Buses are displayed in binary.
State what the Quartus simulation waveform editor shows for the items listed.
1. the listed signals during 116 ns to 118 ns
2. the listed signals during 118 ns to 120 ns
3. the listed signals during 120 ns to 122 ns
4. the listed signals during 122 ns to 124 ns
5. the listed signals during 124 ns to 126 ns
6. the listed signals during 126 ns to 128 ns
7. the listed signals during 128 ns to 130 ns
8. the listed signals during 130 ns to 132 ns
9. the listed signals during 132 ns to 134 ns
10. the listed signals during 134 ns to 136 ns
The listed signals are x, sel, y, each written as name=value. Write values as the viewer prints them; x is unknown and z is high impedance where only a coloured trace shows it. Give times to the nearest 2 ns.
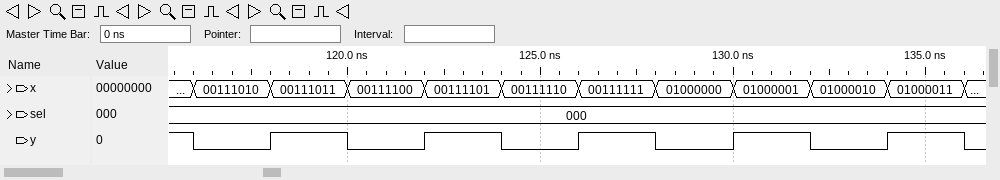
x=00111010, sel=000, y=0
x=00111011, sel=000, y=1
x=00111100, sel=000, y=0
x=00111101, sel=000, y=1
x=00111110, sel=000, y=0
x=00111111, sel=000, y=1
x=01000000, sel=000, y=0
x=01000001, sel=000, y=1
x=01000010, sel=000, y=0
x=01000011, sel=000, y=1
